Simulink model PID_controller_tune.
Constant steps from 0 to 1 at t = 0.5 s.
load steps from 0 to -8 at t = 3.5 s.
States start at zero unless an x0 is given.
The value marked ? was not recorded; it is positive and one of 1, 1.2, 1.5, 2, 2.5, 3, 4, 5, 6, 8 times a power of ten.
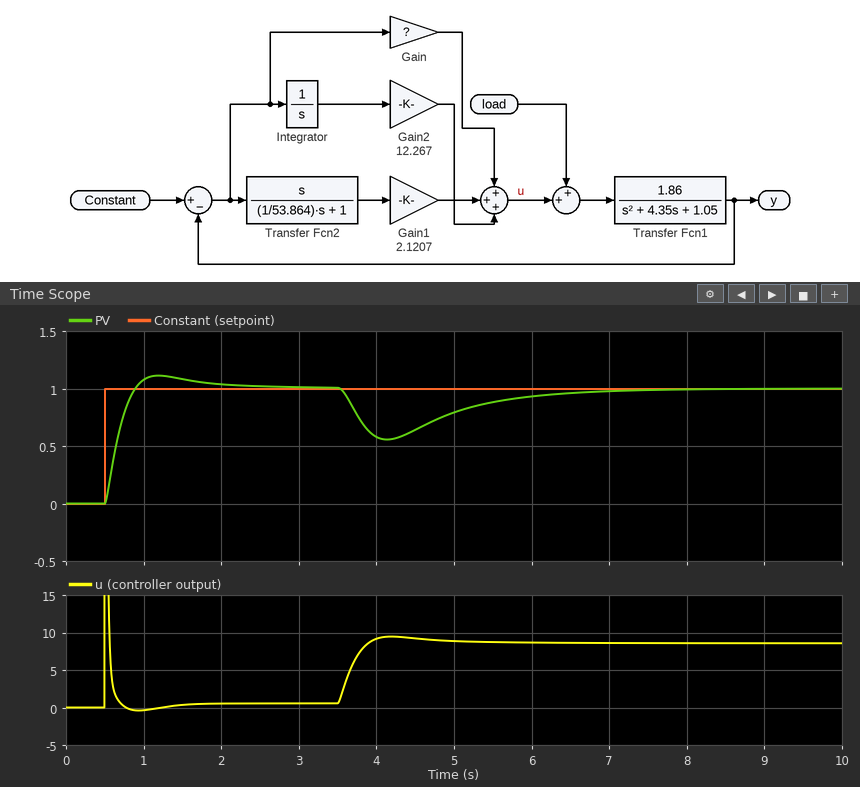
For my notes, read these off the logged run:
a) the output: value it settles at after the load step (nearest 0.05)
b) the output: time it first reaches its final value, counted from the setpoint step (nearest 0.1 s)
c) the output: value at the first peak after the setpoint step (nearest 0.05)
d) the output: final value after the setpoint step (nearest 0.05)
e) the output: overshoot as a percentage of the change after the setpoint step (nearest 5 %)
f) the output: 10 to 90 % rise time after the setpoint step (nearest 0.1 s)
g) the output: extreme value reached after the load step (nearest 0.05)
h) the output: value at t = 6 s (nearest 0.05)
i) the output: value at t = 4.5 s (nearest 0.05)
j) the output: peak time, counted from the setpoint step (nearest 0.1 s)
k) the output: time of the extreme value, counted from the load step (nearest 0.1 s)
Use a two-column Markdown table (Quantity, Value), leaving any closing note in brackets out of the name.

| Quantity | Value |
|---|---|
| the output: value it settles at after the load step | 1.00 |
| the output: time it first reaches its final value, counted from the setpoint step | 0.4 s |
| the output: value at the first peak after the setpoint step | 1.10 |
| the output: final value after the setpoint step | 1.00 |
| the output: overshoot as a percentage of the change after the setpoint step | 10 % |
| the output: 10 to 90 % rise time after the setpoint step | 0.3 s |
| the output: extreme value reached after the load step | 0.55 |
| the output: value at t = 6 s | 0.95 |
| the output: value at t = 4.5 s | 0.65 |
| the output: peak time, counted from the setpoint step | 0.7 s |
| the output: time of the extreme value, counted from the load step | 0.6 s |
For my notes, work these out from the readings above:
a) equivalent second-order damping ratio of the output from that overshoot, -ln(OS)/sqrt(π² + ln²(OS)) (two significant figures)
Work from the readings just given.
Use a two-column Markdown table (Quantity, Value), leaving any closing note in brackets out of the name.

| Quantity | Value |
|---|---|
| equivalent second-order damping ratio of the output from that overshoot, -ln(OS)/sqrt(π² + ln²(OS)) | 0.59 |
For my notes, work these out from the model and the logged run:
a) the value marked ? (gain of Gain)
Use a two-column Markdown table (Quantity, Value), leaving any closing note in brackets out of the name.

| Quantity | Value |
|---|---|
| the value marked ? | 15 |
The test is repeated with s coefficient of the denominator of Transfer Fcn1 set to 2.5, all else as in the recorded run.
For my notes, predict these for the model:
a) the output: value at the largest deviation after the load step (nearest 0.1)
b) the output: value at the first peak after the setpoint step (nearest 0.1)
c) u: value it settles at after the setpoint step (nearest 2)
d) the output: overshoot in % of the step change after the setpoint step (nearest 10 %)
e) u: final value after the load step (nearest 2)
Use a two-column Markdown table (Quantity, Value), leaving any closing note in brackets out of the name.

| Quantity | Value |
|---|---|
| the output: value at the largest deviation after the load step | 0.5 |
| the output: value at the first peak after the setpoint step | 1.2 |
| u: value it settles at after the setpoint step | 0 |
| the output: overshoot in % of the step change after the setpoint step | 20 % |
| u: final value after the load step | 8 |
